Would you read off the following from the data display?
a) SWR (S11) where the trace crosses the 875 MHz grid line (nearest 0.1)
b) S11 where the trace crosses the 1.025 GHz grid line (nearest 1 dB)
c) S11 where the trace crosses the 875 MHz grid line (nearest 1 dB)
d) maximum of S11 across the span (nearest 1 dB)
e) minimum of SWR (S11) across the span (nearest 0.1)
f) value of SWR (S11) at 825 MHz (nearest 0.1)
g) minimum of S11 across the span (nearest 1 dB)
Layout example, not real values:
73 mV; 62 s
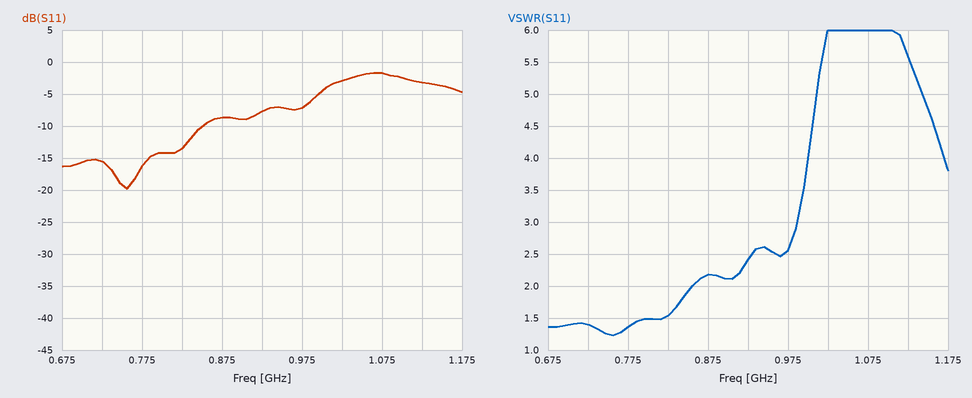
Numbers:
2.2; -3 dB; -9 dB; -2 dB; 1.2; 1.5; -20 dB
